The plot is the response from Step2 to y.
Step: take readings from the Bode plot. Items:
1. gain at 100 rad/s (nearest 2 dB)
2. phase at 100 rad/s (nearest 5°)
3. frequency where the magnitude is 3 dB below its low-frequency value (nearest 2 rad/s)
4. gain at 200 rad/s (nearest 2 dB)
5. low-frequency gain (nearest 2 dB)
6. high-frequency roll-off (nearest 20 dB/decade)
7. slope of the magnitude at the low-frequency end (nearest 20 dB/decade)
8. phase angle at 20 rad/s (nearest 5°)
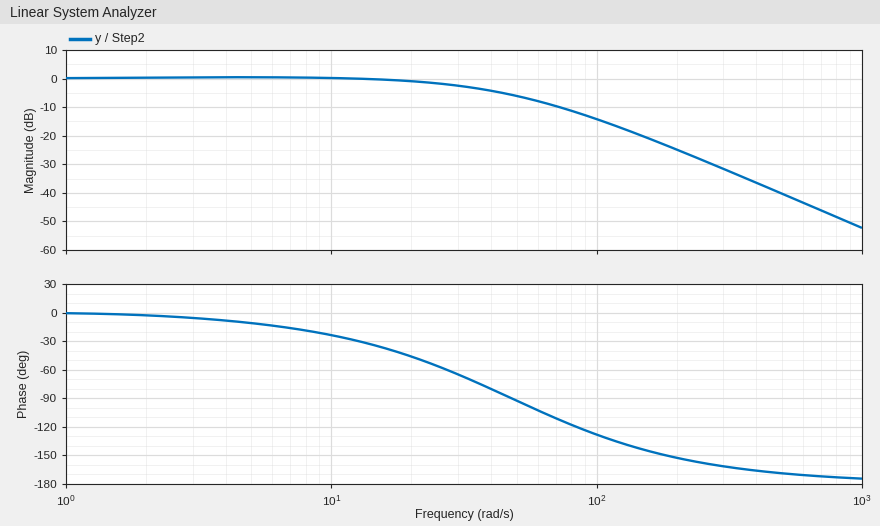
-14 dB
-130°
32 rad/s
-24 dB
0 dB
-40 dB/decade
0 dB/decade
-45°
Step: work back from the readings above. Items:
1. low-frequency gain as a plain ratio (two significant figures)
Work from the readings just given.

1.0
